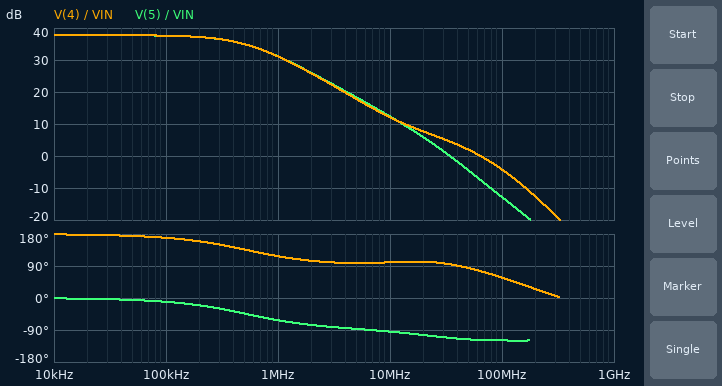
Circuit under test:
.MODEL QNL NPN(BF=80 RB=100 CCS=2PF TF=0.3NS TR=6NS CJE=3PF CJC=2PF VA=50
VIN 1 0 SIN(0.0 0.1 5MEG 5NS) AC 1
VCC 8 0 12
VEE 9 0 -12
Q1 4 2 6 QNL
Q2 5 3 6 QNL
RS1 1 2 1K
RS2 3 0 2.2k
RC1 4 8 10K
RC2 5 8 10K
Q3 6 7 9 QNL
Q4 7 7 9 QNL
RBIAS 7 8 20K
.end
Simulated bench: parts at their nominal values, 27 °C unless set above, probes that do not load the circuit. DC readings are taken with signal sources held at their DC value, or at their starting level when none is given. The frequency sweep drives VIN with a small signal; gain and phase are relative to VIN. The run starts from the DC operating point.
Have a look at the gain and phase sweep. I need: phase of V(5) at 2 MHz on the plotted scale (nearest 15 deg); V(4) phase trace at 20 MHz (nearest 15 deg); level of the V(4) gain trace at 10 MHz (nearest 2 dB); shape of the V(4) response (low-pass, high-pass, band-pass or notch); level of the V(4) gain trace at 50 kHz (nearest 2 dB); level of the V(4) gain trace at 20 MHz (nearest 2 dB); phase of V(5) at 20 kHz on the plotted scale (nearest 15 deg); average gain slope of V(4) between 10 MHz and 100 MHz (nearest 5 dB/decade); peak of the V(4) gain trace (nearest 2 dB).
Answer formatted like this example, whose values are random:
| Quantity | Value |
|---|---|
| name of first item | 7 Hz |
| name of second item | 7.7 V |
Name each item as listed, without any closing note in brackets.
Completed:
| Quantity | Value |
|---|---|
| phase of V(5) at 2 MHz on the plotted scale | -75 deg |
| V(4) phase trace at 20 MHz | 105 deg |
| level of the V(4) gain trace at 10 MHz | 12 dB |
| shape of the V(4) response | low-pass |
| level of the V(4) gain trace at 50 kHz | 38 dB |
| level of the V(4) gain trace at 20 MHz | 8 dB |
| phase of V(5) at 20 kHz on the plotted scale | 0 deg |
| average gain slope of V(4) between 10 MHz and 100 MHz | -15 dB/decade |
| peak of the V(4) gain trace | 38 dB |
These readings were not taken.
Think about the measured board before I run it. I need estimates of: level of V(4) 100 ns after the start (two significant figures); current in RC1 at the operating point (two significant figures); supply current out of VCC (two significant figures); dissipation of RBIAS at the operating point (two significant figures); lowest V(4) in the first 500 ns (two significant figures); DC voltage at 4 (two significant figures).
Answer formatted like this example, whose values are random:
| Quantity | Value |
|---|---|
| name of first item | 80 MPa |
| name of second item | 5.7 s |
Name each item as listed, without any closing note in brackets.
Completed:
| Quantity | Value |
|---|---|
| level of V(4) 100 ns after the start | 3.2 V |
| current in RC1 at the operating point | 750 µA |
| supply current out of VCC | 2.5 mA |
| dissipation of RBIAS at the operating point | 27 mW |
| lowest V(4) in the first 500 ns | 3.2 V |
| DC voltage at 4 | 4.5 V |
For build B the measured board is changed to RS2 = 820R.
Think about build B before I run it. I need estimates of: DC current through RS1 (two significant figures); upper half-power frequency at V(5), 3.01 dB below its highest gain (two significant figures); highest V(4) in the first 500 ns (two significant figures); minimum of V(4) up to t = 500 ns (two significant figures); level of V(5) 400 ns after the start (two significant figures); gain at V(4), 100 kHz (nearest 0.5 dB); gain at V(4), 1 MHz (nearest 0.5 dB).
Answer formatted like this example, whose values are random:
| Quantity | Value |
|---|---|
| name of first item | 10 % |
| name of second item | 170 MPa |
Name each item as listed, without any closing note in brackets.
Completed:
| Quantity | Value |
|---|---|
| DC current through RS1 | 7.5 µA |
| upper half-power frequency at V(5), 3.01 dB below its highest gain | 730 kHz |
| highest V(4) in the first 500 ns | 6.4 V |
| minimum of V(4) up to t = 500 ns | 3.3 V |
| level of V(5) 400 ns after the start | 4.0 V |
| gain at V(4), 100 kHz | 39.0 dB |
| gain at V(4), 1 MHz | 34.5 dB |
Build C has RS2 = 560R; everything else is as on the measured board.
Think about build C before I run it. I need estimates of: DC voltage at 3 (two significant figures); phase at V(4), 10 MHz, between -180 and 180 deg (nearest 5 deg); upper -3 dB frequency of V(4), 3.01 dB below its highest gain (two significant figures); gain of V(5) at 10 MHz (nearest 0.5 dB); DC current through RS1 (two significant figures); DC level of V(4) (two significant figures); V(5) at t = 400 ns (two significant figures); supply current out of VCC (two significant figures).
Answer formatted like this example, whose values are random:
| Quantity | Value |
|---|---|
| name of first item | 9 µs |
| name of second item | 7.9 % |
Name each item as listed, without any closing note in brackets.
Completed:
| Quantity | Value |
|---|---|
| DC voltage at 3 | -4.5 mV |
| phase at V(4), 10 MHz, between -180 and 180 deg | 90 deg |
| upper -3 dB frequency of V(4), 3.01 dB below its highest gain | 800 kHz |
| gain of V(5) at 10 MHz | 17.5 dB |
| DC current through RS1 | 7.3 µA |
| DC level of V(4) | 5.5 V |
| V(5) at t = 400 ns | 3.7 V |
| supply current out of VCC | 2.5 mA |
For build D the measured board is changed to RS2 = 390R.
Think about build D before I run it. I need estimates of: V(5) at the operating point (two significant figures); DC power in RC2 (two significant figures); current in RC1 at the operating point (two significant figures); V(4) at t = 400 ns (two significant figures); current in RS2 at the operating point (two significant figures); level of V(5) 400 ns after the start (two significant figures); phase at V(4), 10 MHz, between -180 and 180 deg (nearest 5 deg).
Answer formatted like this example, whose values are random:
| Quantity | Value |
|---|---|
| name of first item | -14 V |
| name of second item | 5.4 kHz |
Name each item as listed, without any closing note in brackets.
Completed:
| Quantity | Value |
|---|---|
| V(5) at the operating point | 4.8 V |
| DC power in RC2 | 5.2 mW |
| current in RC1 at the operating point | 630 µA |
| V(4) at t = 400 ns | 7.1 V |
| current in RS2 at the operating point | 8.2 µA |
| level of V(5) 400 ns after the start | 3.4 V |
| phase at V(4), 10 MHz, between -180 and 180 deg | 90 deg |
